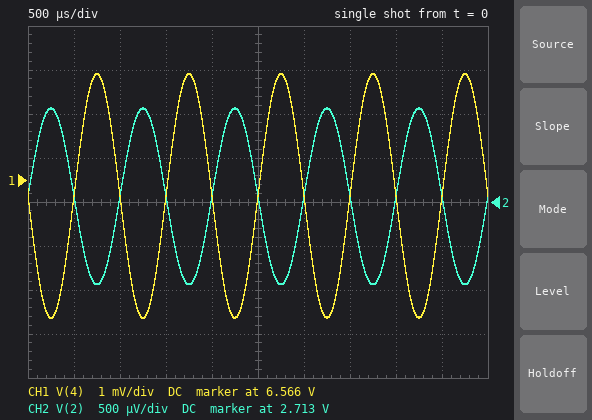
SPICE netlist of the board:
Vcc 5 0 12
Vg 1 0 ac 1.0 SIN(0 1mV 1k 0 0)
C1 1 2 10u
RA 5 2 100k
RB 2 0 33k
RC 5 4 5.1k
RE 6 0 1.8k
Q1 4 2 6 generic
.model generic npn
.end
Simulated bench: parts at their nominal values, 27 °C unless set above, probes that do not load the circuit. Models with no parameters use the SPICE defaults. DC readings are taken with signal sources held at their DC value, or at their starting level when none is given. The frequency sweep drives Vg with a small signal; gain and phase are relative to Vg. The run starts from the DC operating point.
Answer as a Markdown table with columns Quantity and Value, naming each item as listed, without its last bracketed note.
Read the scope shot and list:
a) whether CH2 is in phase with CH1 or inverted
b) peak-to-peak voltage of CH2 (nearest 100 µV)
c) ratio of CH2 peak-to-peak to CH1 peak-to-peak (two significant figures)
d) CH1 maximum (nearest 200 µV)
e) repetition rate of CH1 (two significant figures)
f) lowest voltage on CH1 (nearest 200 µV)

| Quantity | Value |
|---|---|
| whether CH2 is in phase with CH1 or inverted | inverted |
| peak-to-peak voltage of CH2 | 2.0 mV |
| ratio of CH2 peak-to-peak to CH1 peak-to-peak | 0.36 |
| CH1 maximum | 6.5684 V |
| repetition rate of CH1 | 1.0 kHz |
| lowest voltage on CH1 | 6.5628 V |
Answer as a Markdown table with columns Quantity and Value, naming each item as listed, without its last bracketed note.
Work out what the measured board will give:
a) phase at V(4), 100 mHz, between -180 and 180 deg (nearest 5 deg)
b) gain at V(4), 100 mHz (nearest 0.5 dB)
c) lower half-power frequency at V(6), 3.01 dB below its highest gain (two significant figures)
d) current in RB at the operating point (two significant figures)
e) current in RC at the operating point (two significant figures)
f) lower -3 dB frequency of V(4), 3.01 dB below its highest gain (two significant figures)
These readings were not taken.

| Quantity | Value |
|---|---|
| phase at V(4), 100 mHz, between -180 and 180 deg | -100 deg |
| gain at V(4), 100 mHz | -8.5 dB |
| lower half-power frequency at V(6), 3.01 dB below its highest gain | 730 mHz |
| current in RB at the operating point | 82 µA |
| current in RC at the operating point | 1.1 mA |
| lower -3 dB frequency of V(4), 3.01 dB below its highest gain | 730 mHz |
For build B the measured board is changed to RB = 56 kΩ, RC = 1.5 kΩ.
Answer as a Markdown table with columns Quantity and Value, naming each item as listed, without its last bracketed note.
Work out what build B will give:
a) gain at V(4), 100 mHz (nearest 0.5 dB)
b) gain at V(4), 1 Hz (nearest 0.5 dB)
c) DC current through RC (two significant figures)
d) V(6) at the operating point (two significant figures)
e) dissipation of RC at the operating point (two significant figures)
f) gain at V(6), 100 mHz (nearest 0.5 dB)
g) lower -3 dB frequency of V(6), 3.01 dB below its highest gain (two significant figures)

| Quantity | Value |
|---|---|
| gain at V(4), 100 mHz | -16.5 dB |
| gain at V(4), 1 Hz | -3.0 dB |
| DC current through RC | 1.6 mA |
| V(6) at the operating point | 2.9 V |
| dissipation of RC at the operating point | 3.9 mW |
| gain at V(6), 100 mHz | -14.5 dB |
| lower -3 dB frequency of V(6), 3.01 dB below its highest gain | 530 mHz |
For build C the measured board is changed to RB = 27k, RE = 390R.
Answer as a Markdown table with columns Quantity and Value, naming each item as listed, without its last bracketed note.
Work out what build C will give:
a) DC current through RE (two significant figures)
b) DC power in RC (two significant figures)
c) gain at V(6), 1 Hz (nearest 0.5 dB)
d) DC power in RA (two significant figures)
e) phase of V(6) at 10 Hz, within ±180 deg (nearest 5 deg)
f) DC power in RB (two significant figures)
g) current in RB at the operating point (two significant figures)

| Quantity | Value |
|---|---|
| DC current through RE | 2.2 mA |
| DC power in RC | 24 mW |
| gain at V(6), 1 Hz | -31.0 dB |
| DC power in RA | 1.1 mW |
| phase of V(6) at 10 Hz, within ±180 deg | 75 deg |
| DC power in RB | 100 µW |
| current in RB at the operating point | 61 µA |
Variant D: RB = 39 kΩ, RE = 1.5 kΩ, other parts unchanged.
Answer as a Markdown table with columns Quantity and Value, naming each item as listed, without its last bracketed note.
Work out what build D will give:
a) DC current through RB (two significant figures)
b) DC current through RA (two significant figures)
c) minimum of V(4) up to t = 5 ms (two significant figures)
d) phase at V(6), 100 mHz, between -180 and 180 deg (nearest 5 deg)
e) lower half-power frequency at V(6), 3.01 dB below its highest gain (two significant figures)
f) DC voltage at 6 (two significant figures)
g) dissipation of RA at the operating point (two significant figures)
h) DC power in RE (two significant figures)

| Quantity | Value |
|---|---|
| DC current through RB | 76 µA |
| DC current through RA | 90 µA |
| minimum of V(4) up to t = 5 ms | 4.7 V |
| phase at V(6), 100 mHz, between -180 and 180 deg | 80 deg |
| lower half-power frequency at V(6), 3.01 dB below its highest gain | 670 mHz |
| DC voltage at 6 | 2.2 V |
| dissipation of RA at the operating point | 820 µW |
| DC power in RE | 3.2 mW |
